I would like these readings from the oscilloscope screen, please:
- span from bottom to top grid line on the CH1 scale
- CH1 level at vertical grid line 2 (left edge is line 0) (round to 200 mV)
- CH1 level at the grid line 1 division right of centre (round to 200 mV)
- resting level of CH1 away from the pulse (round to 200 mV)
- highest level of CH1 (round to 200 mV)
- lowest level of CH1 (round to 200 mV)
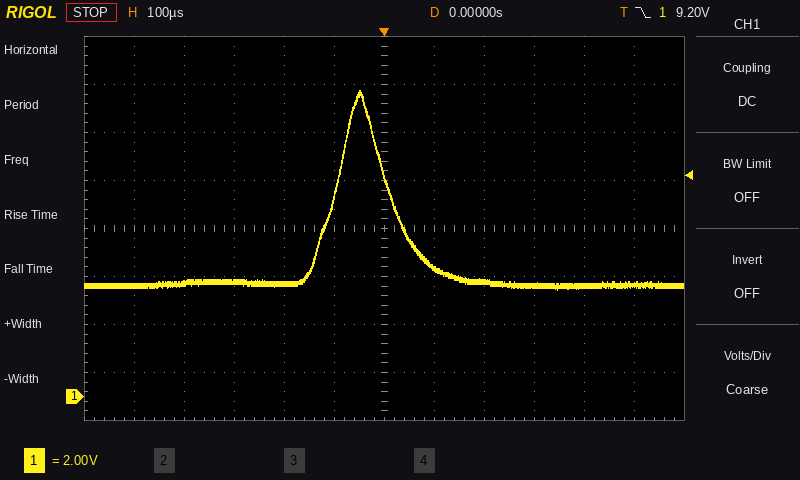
16 V
4.8 V
5.4 V
4.6 V
12.8 V
4.4 V
